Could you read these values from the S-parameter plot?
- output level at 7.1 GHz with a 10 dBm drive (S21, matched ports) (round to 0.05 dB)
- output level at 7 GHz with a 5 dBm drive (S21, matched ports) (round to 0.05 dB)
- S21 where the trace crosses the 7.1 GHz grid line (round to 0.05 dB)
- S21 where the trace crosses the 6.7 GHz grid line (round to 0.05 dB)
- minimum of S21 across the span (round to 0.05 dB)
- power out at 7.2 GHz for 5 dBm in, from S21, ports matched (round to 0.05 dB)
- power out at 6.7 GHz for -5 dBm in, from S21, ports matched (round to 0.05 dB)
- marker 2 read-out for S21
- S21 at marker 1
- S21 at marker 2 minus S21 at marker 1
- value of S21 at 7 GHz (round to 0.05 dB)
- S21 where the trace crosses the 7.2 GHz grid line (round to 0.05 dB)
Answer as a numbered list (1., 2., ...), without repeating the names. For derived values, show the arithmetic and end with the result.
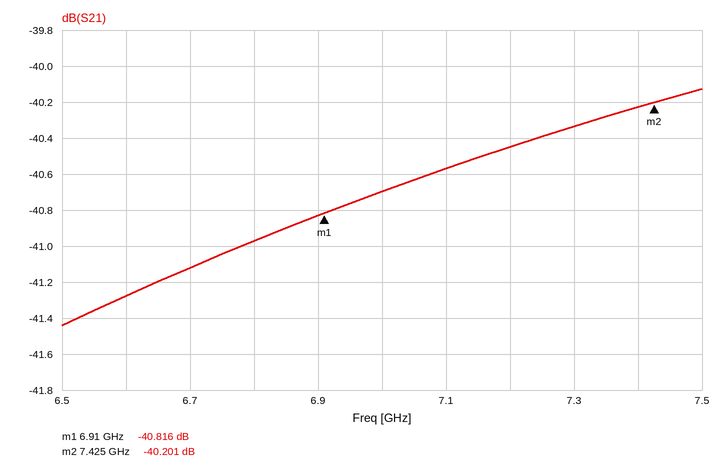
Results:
1. 10 dBm + (-40.55 dB) = -30.55 dBm
2. 5 dBm + (-40.70 dB) = -35.70 dBm
3. -40.55 dB
4. -41.10 dB
5. -41.45 dB
6. 5 dBm + (-40.45 dB) = -35.45 dBm
7. -5 dBm + (-41.10 dB) = -46.10 dBm
8. -40.201 dB
9. -40.816 dB
10. -40.201 − (-40.816) = 0.615 dB
11. -40.70 dB
12. -40.45 dB
